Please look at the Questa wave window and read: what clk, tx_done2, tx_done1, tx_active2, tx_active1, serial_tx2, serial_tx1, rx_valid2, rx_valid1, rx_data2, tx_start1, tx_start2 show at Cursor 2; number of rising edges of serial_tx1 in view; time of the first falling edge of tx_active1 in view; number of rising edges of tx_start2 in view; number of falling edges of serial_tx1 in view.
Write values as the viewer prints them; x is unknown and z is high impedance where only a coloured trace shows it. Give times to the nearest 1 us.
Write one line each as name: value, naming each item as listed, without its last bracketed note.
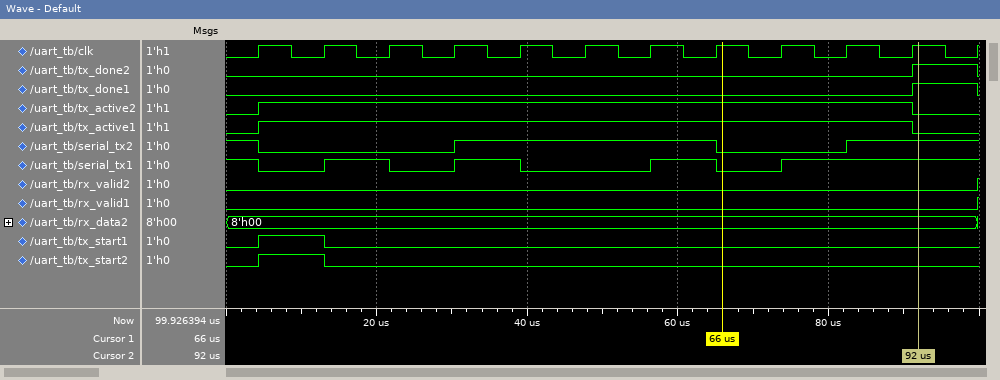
what clk, tx_done2, tx_done1, tx_active2, tx_active1, serial_tx2, serial_tx1, rx_valid2, rx_valid1, rx_data2, tx_start1, tx_start2 show at Cursor 2: clk=1, tx_done2=1, tx_done1=1, tx_active2=0, tx_active1=0, serial_tx2=1, serial_tx1=1, rx_valid2=0, rx_valid1=0, rx_data2=8'h00, tx_start1=0, tx_start2=0
number of rising edges of serial_tx1 in view: 4
time of the first falling edge of tx_active1 in view: 91 us
number of rising edges of tx_start2 in view: 1
number of falling edges of serial_tx1 in view: 4
